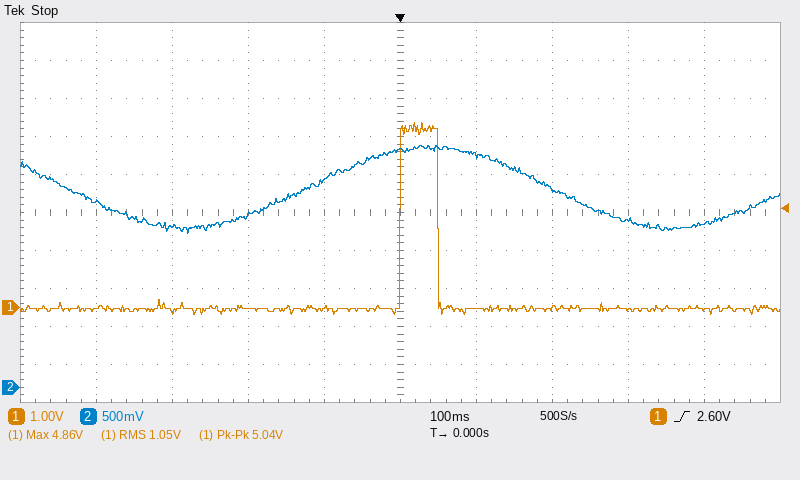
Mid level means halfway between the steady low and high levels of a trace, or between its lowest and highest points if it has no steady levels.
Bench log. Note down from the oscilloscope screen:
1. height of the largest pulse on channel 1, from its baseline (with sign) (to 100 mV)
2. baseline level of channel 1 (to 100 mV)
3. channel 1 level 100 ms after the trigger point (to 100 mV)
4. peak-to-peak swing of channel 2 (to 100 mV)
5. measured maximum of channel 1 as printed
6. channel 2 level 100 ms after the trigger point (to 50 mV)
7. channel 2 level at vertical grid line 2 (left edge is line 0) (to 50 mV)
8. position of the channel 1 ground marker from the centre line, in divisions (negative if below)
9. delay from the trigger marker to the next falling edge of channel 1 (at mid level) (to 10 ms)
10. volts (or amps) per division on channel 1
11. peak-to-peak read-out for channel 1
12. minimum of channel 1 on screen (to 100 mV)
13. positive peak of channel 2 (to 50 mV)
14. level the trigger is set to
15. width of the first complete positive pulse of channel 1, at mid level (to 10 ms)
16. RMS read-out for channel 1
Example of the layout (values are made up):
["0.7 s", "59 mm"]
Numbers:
["+4.9 V", "0.0 V", "0.0 V", "1.20 V", "4.86 V", "3.05 V", "2.10 V", "-2.5 div", "50 ms", "1 V", "5.04 V", "-200 mV", "3.20 V", "2.60 V", "50 ms", "1.05 V"]
